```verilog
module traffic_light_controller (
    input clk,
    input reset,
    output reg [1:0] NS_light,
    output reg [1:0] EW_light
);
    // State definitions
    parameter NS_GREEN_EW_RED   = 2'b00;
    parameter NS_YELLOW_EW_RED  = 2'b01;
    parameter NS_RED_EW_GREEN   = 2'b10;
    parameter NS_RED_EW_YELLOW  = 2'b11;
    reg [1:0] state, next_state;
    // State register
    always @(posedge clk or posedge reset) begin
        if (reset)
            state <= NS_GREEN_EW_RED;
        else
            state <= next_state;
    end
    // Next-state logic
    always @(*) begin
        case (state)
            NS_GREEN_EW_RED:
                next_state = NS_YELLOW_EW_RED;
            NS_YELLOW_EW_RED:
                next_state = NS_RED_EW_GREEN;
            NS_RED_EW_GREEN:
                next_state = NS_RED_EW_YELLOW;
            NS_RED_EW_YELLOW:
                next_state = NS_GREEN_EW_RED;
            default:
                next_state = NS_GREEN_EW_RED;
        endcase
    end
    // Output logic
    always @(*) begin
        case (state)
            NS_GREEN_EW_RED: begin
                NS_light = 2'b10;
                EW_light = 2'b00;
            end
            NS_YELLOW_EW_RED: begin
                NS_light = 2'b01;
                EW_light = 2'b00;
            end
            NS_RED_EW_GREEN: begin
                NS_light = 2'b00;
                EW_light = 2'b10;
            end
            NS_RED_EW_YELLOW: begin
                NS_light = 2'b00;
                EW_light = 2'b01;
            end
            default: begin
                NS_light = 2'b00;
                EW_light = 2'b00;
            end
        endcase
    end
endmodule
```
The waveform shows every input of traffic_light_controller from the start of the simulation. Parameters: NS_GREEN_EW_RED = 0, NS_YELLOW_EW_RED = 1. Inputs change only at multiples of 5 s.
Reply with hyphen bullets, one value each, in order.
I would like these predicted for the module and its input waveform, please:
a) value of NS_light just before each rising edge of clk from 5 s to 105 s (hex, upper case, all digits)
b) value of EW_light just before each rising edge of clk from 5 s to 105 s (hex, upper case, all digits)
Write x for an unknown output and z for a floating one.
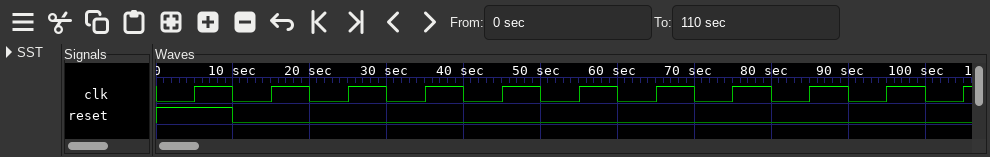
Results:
- 2, 2, 1, 0, 0, 2, 1, 0, 0, 2, 1
- 0, 0, 0, 2, 1, 0, 0, 2, 1, 0, 0
